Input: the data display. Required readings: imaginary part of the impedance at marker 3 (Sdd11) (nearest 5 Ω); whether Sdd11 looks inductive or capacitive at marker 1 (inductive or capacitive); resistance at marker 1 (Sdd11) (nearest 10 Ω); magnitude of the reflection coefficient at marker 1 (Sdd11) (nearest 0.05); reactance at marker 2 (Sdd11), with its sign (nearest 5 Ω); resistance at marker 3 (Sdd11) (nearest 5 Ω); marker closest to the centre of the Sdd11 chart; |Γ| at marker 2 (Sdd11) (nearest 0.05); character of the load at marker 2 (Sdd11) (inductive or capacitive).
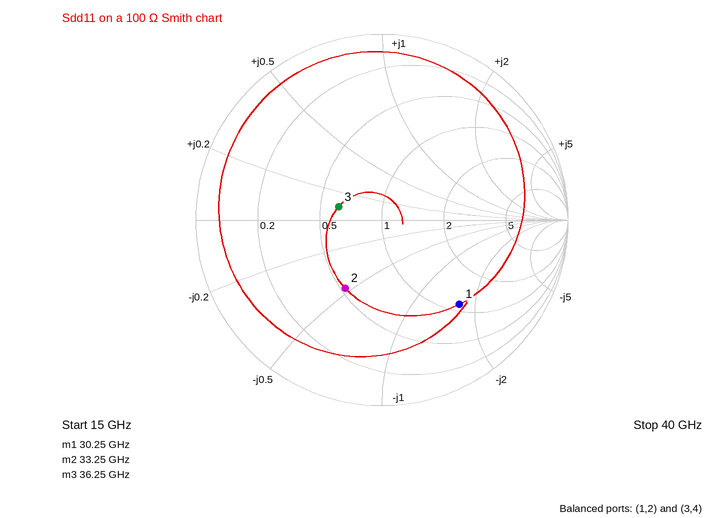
+10 Ω
capacitive
110 Ω
0.60
-45 Ω
60 Ω
marker 3
0.40
capacitive
